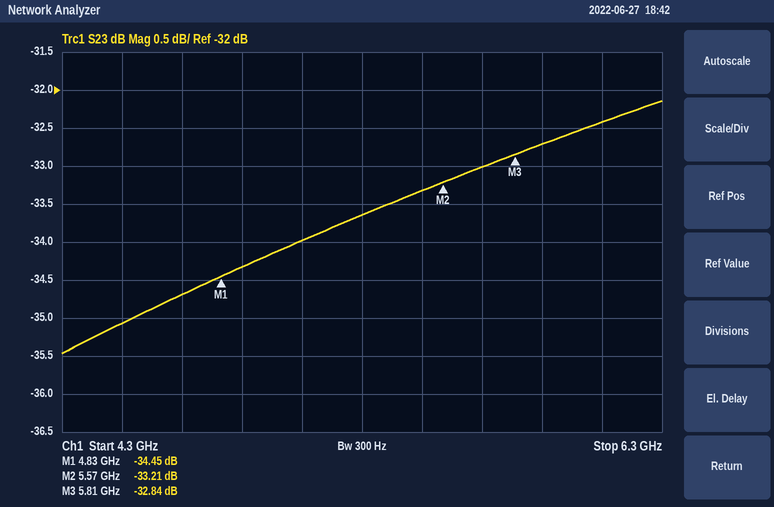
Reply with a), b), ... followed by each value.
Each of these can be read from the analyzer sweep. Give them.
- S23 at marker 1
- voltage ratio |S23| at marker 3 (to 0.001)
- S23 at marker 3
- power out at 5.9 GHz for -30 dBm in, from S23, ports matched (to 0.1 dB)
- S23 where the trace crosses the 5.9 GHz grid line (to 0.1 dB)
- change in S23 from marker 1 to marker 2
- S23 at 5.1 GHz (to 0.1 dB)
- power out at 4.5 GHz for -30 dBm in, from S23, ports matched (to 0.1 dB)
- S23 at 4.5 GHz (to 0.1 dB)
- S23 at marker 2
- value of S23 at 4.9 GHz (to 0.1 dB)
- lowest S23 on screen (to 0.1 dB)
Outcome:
a) -34.45 dB
b) 0.023
c) -32.84 dB
d) -62.7 dBm
e) -32.7 dB
f) 1.24 dB
g) -34.0 dB
h) -65.1 dBm
i) -35.1 dB
j) -33.21 dB
k) -34.3 dB
l) -35.5 dB
